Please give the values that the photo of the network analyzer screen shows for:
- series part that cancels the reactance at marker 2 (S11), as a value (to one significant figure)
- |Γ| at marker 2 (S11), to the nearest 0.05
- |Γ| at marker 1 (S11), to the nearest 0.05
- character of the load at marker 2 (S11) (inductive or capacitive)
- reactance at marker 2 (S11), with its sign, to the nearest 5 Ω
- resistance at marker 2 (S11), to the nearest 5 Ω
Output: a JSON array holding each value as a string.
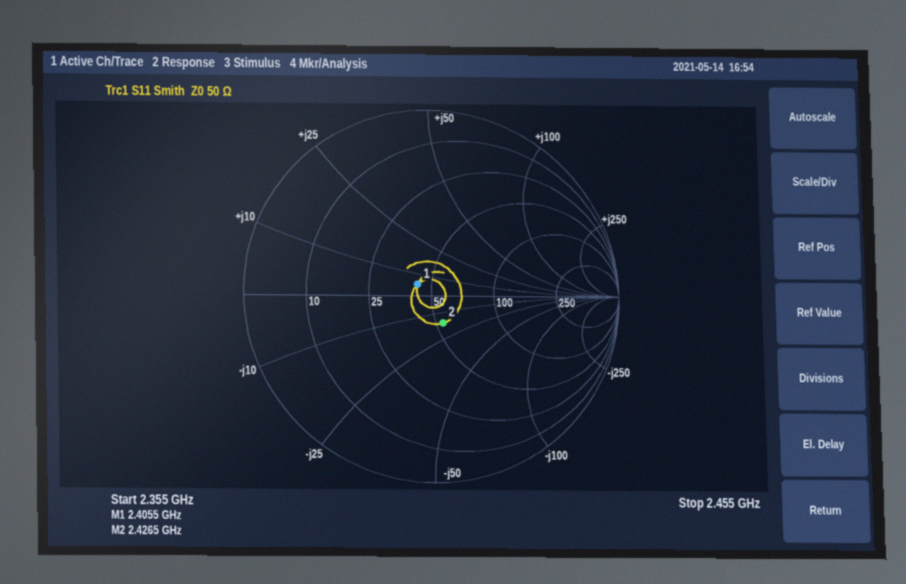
["1 nH", "0.15", "0.10", "capacitive", "-15 Ω", "55 Ω"]
